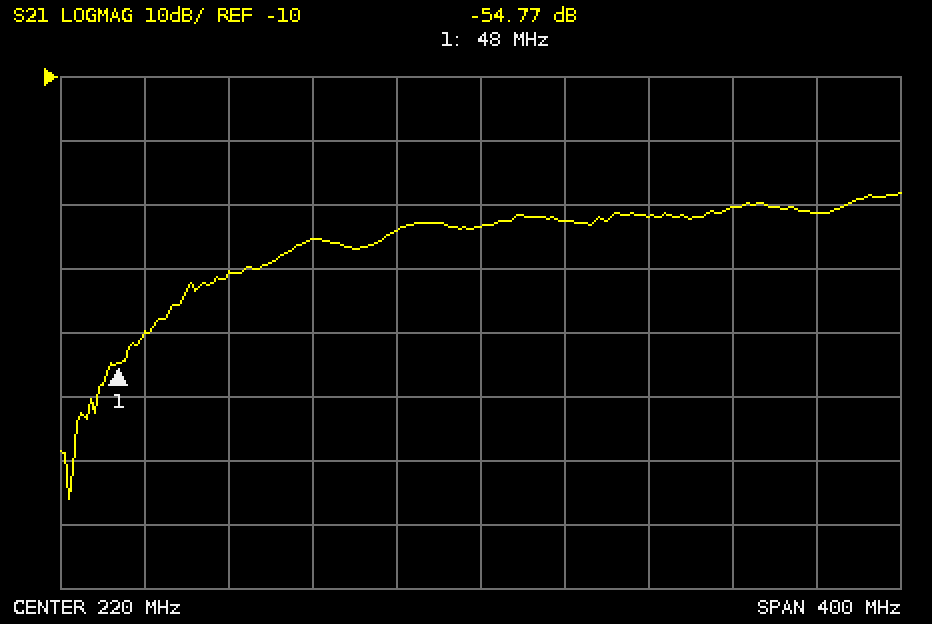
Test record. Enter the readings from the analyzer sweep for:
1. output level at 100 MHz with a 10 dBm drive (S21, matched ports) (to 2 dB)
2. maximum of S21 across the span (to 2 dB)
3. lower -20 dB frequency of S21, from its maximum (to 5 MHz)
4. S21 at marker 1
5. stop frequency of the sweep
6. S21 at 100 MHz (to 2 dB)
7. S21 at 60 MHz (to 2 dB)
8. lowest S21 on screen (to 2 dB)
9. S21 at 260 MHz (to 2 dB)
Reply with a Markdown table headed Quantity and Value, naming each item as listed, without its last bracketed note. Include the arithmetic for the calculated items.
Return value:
| Quantity | Value |
|---|---|
| output level at 100 MHz with a 10 dBm drive (S21, matched ports) | 10 dBm + (-40 dB) = -30 dBm |
| maximum of S21 across the span | -28 dB |
| lower -20 dB frequency of S21, from its maximum | 65 MHz |
| S21 at marker 1 | -54.77 dB |
| stop frequency of the sweep | 420 MHz |
| S21 at 100 MHz | -40 dB |
| S21 at 60 MHz | -50 dB |
| lowest S21 on screen | -76 dB |
| S21 at 260 MHz | -32 dB |
